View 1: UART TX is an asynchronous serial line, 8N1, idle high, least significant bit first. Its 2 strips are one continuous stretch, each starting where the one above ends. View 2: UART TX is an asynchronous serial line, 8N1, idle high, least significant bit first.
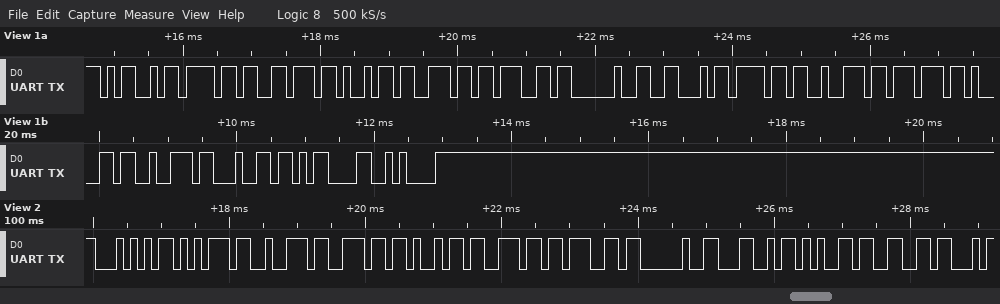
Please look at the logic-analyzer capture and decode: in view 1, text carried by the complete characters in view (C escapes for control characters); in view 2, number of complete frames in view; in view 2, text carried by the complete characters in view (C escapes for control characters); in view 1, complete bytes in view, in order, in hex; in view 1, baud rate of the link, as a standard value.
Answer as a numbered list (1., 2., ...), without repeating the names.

1. "Moving Forward\r\n"
2. 11
3. "Turning Lef"
4. 0x4D 0x6F 0x76 0x69 0x6E 0x67 0x20 0x46 0x6F 0x72 0x77 0x61 0x72 0x64 0x0D 0x0A
5. 9600 baud
